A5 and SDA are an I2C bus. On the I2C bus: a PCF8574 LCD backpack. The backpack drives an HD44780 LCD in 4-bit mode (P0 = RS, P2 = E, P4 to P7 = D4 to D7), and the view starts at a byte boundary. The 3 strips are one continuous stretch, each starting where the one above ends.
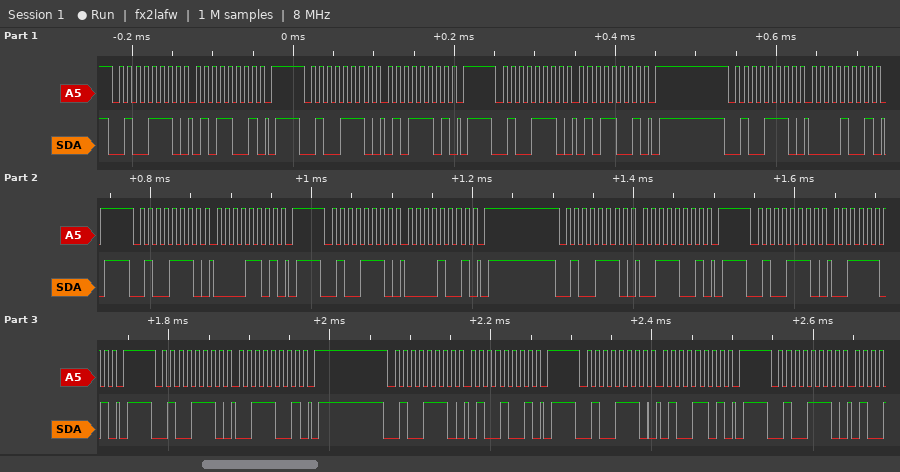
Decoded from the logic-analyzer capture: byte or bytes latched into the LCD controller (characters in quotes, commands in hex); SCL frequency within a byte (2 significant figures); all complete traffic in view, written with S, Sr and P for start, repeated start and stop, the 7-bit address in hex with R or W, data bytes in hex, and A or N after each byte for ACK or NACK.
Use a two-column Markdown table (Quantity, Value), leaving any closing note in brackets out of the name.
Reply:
| Quantity | Value |
|---|---|
| byte or bytes latched into the LCD controller | 'P' |
| SCL frequency within a byte | 100 kHz |
| all complete traffic in view, written with S, Sr and P for start, repeated start and stop, the 7-bit address in hex with R or W, data bytes in hex, and A or N after each byte for ACK or NACK | S 27W A 59 A P S 27W A 5D A P S 27W A 59 A P S 27W A 09 A P S 27W A 0D A P S 27W A 09 A P S 27W A 39 A P S 27W A 3D A P S 27W A 39 A P S 27W A 49 A P S 27W A 4D A P S 27W A |
